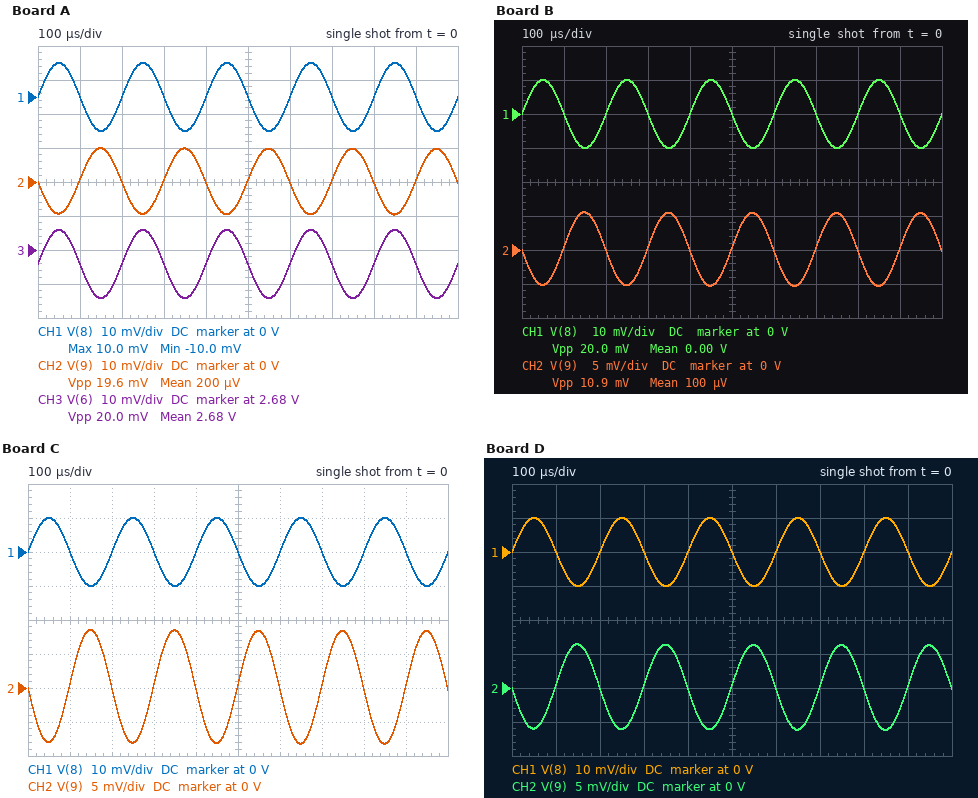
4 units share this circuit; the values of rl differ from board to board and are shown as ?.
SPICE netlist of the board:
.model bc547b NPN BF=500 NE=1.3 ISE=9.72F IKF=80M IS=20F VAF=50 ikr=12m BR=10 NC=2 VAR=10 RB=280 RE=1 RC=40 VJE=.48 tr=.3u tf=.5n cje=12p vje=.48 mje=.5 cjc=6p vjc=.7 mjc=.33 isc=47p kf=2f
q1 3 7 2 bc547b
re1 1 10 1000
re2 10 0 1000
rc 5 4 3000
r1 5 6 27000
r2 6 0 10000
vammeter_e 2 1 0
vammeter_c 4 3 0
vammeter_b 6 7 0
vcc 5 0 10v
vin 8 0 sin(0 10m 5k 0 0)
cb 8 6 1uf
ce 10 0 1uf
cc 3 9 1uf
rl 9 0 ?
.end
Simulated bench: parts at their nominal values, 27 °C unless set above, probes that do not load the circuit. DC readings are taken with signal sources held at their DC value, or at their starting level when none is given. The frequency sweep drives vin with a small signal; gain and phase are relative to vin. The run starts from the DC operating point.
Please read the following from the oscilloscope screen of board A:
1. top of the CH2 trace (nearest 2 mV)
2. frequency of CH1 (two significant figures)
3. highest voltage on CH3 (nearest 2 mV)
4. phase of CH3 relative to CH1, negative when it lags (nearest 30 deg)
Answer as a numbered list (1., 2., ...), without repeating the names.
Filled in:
1. 10 mV
2. 5.0 kHz
3. 2.686 V
4. 0 deg
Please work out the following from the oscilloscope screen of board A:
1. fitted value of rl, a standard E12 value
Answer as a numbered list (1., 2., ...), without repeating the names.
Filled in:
1. 1.5 kΩ
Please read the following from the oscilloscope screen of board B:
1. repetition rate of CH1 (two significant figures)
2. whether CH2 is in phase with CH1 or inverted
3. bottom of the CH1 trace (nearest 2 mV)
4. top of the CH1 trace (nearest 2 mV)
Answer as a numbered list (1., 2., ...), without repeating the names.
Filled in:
1. 5.0 kHz
2. inverted
3. -10 mV
4. 10 mV
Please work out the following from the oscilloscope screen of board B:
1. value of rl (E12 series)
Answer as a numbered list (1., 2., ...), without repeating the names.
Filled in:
1. 680 Ω
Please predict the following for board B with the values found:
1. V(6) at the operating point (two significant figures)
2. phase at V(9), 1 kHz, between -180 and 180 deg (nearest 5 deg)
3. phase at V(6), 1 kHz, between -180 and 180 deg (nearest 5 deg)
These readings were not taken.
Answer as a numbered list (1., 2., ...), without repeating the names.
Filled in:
1. 2.7 V
2. -170 deg
3. 0 deg
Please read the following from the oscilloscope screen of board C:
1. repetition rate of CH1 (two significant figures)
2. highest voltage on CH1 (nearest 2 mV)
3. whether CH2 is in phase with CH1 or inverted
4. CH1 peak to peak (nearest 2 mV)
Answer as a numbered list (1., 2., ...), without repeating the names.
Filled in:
1. 5.0 kHz
2. 10 mV
3. inverted
4. 20 mV
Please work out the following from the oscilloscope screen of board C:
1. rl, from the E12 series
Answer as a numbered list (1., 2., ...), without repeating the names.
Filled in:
1. 1.2 kΩ
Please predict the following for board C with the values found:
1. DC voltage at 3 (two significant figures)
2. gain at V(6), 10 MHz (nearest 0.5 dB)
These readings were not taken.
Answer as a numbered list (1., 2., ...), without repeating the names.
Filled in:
1. 7.0 V
2. 0 dB
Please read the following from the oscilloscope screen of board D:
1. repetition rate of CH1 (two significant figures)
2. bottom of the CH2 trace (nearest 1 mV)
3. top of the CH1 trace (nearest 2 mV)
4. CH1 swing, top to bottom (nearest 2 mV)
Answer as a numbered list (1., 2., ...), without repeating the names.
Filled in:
1. 5.0 kHz
2. -6 mV
3. 10 mV
4. 20 mV
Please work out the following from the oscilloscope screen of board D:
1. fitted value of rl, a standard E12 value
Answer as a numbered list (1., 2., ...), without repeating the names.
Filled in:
1. 820 Ω
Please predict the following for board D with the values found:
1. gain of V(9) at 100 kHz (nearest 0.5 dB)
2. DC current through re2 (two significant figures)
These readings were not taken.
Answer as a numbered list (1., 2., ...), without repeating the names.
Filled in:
1. -4.0 dB
2. 1.0 mA
